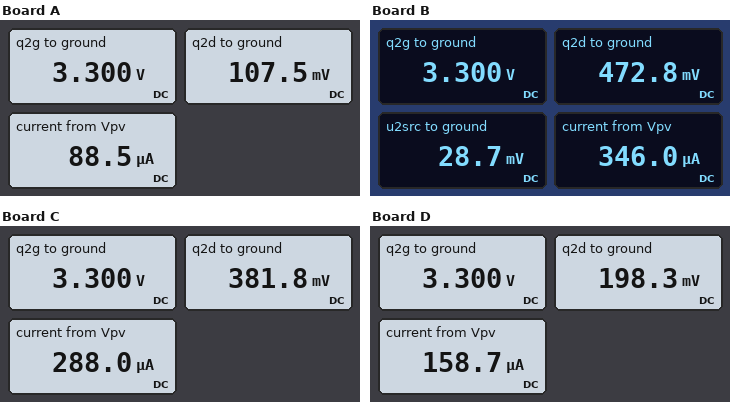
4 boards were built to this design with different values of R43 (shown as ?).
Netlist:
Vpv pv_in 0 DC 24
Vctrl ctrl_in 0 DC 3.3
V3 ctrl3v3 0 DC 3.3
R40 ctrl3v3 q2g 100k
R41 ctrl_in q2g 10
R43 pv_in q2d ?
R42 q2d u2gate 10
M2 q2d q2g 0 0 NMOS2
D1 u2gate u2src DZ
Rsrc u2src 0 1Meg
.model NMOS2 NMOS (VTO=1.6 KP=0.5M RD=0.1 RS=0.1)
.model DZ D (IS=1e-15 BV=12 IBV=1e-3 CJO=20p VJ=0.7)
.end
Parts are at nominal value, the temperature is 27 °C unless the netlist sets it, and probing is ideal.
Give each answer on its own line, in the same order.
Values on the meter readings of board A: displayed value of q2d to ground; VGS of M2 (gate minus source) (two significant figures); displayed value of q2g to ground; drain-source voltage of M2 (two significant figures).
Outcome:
107.5 mV
3.3 V
3.300 V
110 mV
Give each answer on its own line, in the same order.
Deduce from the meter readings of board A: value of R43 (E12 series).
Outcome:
270 kΩ
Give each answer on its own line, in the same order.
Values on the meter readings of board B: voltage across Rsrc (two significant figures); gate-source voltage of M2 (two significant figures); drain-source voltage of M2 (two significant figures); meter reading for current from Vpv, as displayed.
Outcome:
29 mV
3.3 V
470 mV
346.0 µA
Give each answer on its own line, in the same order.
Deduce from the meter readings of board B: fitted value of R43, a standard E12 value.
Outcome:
68 kΩ
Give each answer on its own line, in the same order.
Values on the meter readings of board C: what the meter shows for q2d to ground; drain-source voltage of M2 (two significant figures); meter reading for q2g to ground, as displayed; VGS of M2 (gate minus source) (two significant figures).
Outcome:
381.8 mV
380 mV
3.300 V
3.3 V
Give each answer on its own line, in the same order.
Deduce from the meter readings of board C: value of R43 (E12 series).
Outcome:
82 kΩ
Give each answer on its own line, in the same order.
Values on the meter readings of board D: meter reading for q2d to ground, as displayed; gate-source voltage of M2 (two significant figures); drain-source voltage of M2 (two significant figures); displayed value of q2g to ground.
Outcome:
198.3 mV
3.3 V
200 mV
3.300 V
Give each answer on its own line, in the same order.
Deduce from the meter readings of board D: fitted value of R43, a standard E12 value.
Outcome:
150 kΩ
